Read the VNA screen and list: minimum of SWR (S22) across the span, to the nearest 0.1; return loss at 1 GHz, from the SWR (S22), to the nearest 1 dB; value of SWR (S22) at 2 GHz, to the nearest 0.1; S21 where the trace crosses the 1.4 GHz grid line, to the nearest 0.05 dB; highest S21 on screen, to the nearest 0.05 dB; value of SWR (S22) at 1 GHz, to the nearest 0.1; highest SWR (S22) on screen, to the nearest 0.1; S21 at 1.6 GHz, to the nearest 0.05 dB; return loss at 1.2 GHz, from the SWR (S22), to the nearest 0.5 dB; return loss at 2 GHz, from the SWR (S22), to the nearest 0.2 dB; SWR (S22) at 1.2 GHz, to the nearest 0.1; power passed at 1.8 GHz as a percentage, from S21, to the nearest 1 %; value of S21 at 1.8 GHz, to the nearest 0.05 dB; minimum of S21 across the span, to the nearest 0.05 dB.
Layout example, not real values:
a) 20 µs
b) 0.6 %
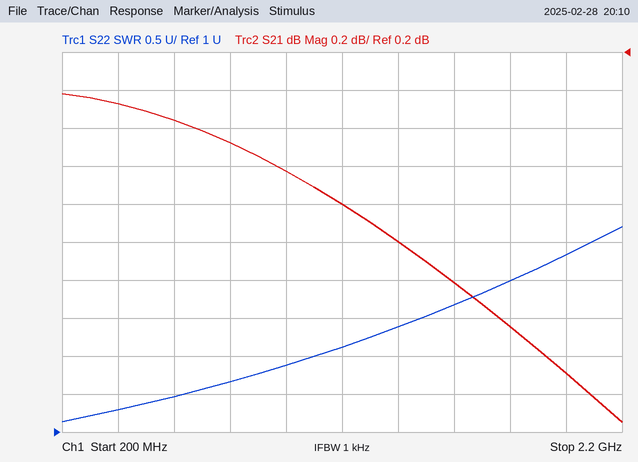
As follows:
a) 1.1
b) 10 dB
c) 3.3
d) -0.80 dB
e) 0.00 dB
f) 1.9
g) 3.7
h) -1.00 dB
i) 9.0 dB
j) 5.4 dB
k) 2.1
l) 75 %
m) -1.25 dB
n) -1.75 dB
